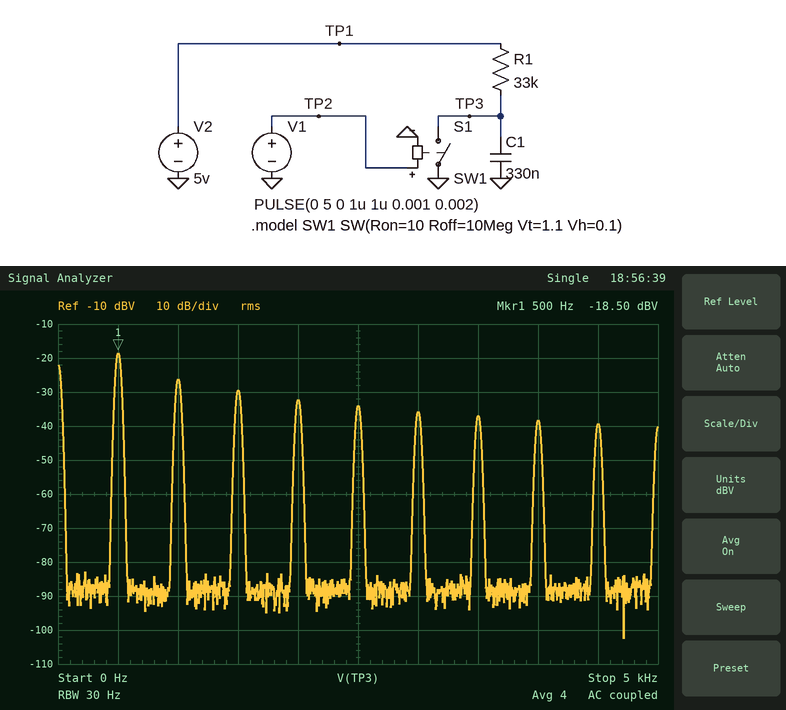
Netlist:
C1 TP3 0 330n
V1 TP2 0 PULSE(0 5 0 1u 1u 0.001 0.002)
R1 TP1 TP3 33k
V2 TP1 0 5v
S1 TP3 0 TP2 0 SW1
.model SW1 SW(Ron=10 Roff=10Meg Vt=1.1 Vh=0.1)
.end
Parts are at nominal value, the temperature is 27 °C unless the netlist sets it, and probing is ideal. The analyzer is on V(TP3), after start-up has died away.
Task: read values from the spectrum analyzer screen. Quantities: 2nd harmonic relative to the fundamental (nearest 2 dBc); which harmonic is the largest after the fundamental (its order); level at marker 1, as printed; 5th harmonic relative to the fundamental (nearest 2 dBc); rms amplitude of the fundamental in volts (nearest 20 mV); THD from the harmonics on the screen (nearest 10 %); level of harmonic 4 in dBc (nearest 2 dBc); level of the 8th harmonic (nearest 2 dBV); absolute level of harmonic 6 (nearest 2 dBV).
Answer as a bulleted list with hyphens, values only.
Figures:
- -8 dBc
- 2
- -18.50 dBV
- -16 dBc
- 120 mV
- 60 %
- -14 dBc
- -38 dBV
- -36 dBV
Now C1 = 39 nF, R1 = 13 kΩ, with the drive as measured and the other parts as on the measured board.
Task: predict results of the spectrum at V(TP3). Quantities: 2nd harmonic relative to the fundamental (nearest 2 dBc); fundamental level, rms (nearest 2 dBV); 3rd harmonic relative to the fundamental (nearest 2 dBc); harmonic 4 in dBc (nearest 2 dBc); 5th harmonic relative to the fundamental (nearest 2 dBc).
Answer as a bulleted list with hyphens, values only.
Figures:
- -10 dBc
- 4 dBV
- -12 dBc
- -16 dBc
- -18 dBc
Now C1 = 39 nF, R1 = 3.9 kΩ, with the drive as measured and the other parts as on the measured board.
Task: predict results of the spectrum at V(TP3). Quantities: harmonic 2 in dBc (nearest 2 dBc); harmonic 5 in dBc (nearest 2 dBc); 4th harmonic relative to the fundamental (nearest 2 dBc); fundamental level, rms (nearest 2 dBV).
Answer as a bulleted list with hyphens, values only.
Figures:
- -14 dBc
- -18 dBc
- -18 dBc
- 6 dBV
